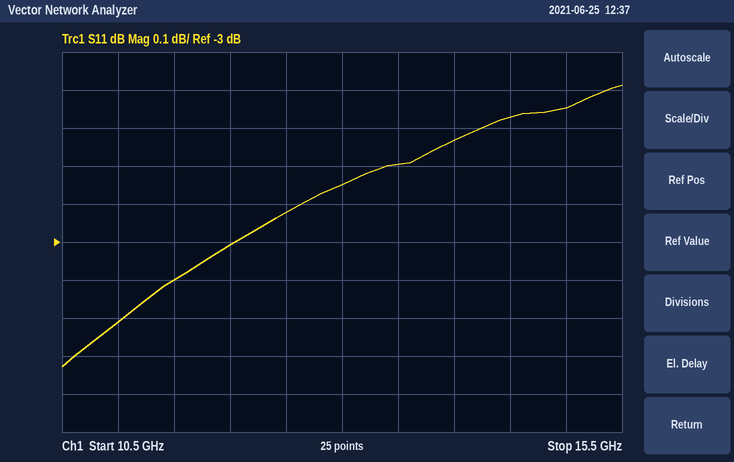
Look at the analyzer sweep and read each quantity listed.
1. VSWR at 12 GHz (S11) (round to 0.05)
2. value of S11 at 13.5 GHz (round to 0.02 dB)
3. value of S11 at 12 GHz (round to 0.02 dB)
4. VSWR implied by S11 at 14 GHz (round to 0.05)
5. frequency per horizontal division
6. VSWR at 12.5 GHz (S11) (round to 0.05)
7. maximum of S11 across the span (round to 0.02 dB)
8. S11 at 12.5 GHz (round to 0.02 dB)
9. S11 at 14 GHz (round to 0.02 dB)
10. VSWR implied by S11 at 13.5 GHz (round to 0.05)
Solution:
5.85
-2.80 dB
-3.00 dB
6.40
500 MHz
6.00
-2.58 dB
-2.92 dB
-2.74 dB
6.25
